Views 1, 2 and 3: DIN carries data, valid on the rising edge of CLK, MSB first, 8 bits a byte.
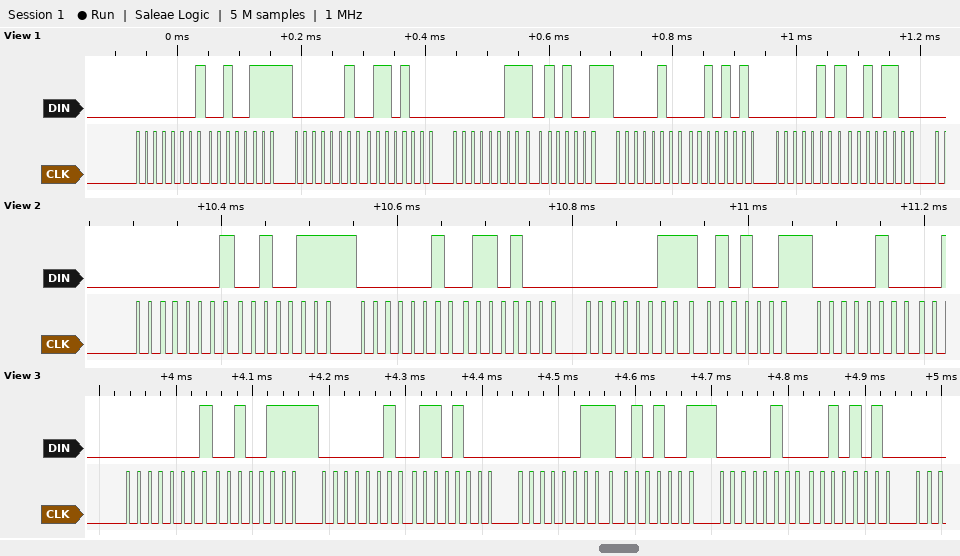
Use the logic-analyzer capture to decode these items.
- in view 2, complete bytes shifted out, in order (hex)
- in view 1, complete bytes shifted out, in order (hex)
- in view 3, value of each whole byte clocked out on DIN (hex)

01 27 02 68 03 A9 04
01 27 02 68 03 A9 04 2A 05 2C
01 27 02 68 03 A9 04 2A
